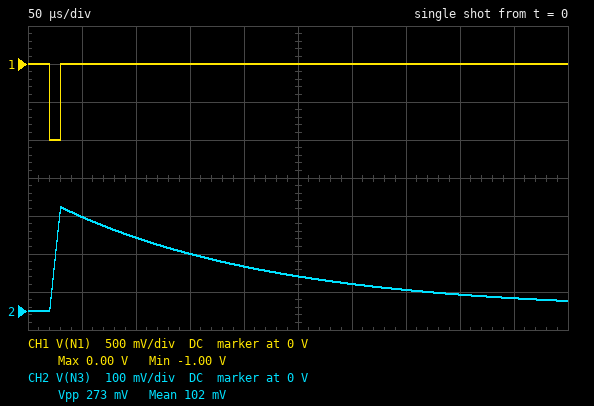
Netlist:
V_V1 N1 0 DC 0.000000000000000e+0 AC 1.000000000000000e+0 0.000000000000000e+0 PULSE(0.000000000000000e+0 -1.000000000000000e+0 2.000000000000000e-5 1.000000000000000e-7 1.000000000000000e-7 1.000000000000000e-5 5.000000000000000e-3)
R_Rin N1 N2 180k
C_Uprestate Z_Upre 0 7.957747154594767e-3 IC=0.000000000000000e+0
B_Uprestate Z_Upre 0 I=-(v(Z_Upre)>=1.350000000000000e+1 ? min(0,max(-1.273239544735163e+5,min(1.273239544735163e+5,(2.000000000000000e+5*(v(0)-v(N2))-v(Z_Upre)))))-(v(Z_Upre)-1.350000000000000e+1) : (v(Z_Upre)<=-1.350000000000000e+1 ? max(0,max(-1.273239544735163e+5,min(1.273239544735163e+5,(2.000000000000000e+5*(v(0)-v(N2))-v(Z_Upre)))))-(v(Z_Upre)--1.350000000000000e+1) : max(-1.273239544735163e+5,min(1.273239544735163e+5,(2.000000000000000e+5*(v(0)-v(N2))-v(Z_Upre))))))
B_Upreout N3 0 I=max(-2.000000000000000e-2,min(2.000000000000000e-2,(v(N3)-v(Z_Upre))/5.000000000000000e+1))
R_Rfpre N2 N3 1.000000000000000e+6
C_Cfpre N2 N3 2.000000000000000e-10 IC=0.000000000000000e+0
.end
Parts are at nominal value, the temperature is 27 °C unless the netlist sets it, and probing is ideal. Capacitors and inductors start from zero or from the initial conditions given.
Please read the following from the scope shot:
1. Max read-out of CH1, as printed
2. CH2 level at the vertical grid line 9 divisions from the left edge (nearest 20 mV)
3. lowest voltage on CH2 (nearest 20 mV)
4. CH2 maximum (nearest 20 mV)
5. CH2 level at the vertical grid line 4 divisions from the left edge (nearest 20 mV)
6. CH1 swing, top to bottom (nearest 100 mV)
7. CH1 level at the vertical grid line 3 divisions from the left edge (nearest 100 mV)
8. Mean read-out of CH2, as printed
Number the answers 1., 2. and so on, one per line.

1. 0.00 V
2. 40 mV
3. 0 V
4. 280 mV
5. 120 mV
6. 1.0 V
7. 0 V
8. 102 mV
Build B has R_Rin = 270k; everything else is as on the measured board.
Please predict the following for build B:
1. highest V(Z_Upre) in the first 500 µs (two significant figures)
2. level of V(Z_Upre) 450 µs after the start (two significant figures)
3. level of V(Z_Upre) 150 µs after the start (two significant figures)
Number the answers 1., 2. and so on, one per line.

1. 180 mV
2. 22 mV
3. 100 mV
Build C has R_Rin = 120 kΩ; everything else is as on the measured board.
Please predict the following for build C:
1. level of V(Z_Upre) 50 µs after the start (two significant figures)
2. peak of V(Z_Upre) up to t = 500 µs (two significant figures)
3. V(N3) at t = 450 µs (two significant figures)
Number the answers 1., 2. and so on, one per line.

1. 370 mV
2. 410 mV
3. 50 mV
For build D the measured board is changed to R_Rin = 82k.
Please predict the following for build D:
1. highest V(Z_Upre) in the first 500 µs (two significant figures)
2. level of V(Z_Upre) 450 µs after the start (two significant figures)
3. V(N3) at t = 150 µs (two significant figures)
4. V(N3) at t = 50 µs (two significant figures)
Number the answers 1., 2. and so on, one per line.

1. 600 mV
2. 74 mV
3. 330 mV
4. 540 mV
